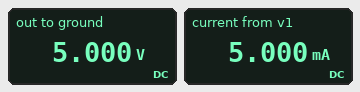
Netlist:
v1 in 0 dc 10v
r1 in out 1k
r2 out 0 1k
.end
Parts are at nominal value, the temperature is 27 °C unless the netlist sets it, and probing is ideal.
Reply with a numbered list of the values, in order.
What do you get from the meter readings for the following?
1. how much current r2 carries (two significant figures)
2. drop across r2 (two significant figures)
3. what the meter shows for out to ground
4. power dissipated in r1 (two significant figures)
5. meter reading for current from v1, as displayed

1. 5.0 mA
2. 5.0 V
3. 5.000 V
4. 25 mW
5. 5.000 mA
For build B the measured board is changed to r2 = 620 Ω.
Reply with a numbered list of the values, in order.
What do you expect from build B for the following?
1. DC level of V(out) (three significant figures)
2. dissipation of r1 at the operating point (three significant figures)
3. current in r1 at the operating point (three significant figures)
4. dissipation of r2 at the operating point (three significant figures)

1. 3.83 V
2. 38.1 mW
3. 6.17 mA
4. 23.6 mW
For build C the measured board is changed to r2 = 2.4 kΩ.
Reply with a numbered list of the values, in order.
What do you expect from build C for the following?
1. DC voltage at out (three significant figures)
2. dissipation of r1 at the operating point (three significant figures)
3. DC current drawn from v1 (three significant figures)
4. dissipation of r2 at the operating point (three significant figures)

1. 7.06 V
2. 8.65 mW
3. 2.94 mA
4. 20.8 mW
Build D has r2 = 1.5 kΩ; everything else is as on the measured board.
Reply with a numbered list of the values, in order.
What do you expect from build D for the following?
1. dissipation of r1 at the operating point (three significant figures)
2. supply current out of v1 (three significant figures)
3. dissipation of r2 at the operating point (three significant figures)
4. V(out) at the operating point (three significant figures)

1. 16.0 mW
2. 4.00 mA
3. 24.0 mW
4. 6.00 V
